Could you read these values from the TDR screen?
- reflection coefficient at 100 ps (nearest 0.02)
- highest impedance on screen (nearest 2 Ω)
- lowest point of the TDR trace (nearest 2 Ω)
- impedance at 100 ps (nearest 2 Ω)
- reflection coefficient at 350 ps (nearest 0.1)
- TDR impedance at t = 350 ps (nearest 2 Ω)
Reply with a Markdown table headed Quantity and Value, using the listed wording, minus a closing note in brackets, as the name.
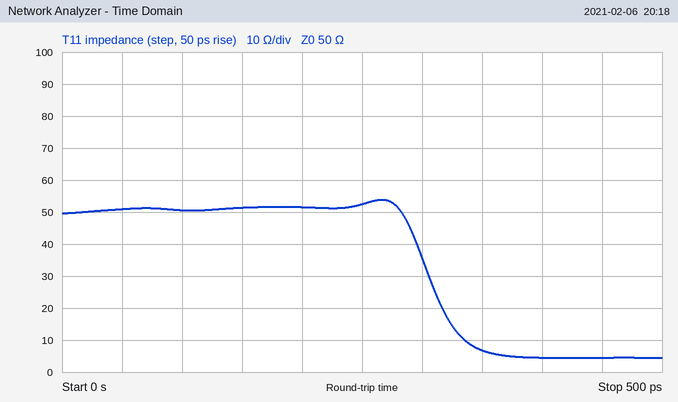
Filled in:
| Quantity | Value |
|---|---|
| reflection coefficient at 100 ps | 0.00 |
| highest impedance on screen | 54 Ω |
| lowest point of the TDR trace | 4 Ω |
| impedance at 100 ps | 50 Ω |
| reflection coefficient at 350 ps | -0.8 |
| TDR impedance at t = 350 ps | 6 Ω |
